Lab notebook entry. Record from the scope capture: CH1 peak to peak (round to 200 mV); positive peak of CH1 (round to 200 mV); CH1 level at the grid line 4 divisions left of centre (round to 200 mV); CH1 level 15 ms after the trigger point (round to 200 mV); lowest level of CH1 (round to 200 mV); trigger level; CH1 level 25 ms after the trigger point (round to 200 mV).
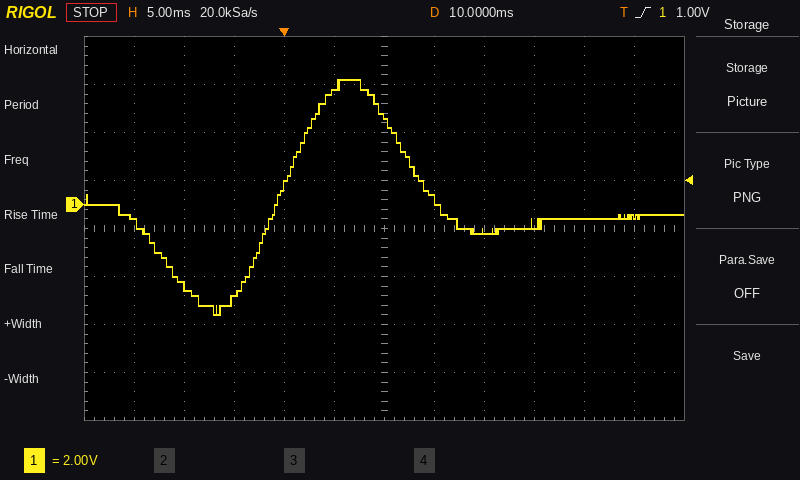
9.8 V
5.2 V
-3.4 V
200 mV
-4.6 V
1.00 V
-800 mV
